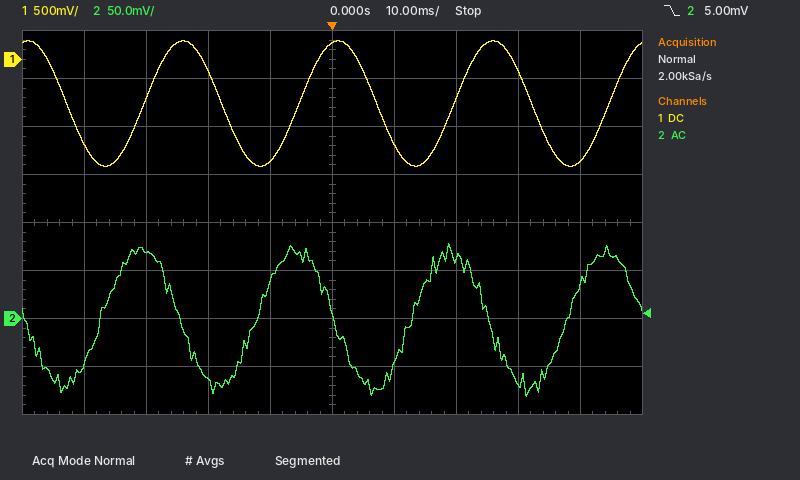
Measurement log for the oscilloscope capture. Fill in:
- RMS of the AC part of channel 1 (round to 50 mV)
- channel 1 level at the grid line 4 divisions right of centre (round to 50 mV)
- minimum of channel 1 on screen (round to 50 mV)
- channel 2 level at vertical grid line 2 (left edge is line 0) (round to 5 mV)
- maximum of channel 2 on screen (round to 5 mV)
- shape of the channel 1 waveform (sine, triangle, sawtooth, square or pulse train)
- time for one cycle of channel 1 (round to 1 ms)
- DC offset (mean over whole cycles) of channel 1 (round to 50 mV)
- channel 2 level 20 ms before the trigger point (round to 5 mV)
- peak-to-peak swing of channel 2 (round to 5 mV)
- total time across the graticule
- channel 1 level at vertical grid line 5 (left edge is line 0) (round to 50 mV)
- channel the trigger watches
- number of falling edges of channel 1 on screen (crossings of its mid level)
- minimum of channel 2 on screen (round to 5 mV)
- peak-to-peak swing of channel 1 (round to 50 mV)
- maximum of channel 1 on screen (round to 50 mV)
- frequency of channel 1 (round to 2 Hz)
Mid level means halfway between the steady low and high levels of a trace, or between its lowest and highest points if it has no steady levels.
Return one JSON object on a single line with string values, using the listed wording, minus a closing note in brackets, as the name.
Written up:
{"RMS of the AC part of channel 1": "450 mV", "channel 1 level at the grid line 4 divisions right of centre": "-1.05 V", "minimum of channel 1 on screen": "-1.10 V", "channel 2 level at vertical grid line 2 (left edge is line 0)": "70 mV", "maximum of channel 2 on screen": "80 mV", "shape of the channel 1 waveform": "sine", "time for one cycle of channel 1": "25 ms", "DC offset (mean over whole cycles) of channel 1": "-450 mV", "channel 2 level 20 ms before the trigger point": "-65 mV", "peak-to-peak swing of channel 2": "160 mV", "total time across the graticule": "100 ms", "channel 1 level at vertical grid line 5 (left edge is line 0)": "150 mV", "channel the trigger watches": "channel 2", "number of falling edges of channel 1 on screen": "4", "minimum of channel 2 on screen": "-80 mV", "peak-to-peak swing of channel 1": "1.30 V", "maximum of channel 1 on screen": "200 mV", "frequency of channel 1": "40 Hz"}
